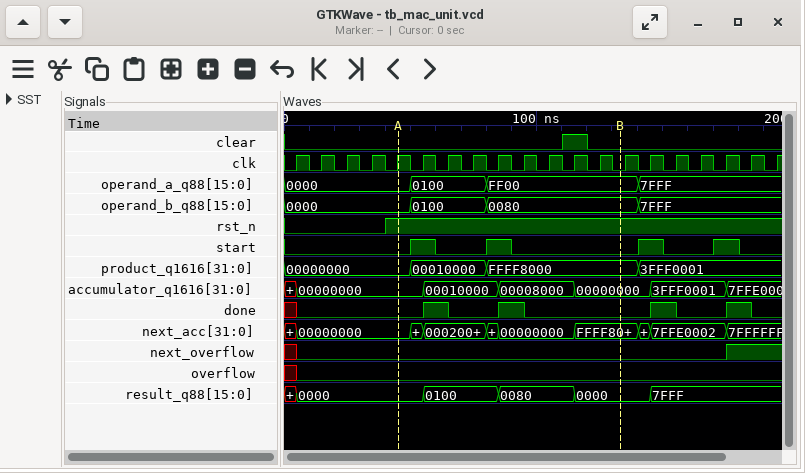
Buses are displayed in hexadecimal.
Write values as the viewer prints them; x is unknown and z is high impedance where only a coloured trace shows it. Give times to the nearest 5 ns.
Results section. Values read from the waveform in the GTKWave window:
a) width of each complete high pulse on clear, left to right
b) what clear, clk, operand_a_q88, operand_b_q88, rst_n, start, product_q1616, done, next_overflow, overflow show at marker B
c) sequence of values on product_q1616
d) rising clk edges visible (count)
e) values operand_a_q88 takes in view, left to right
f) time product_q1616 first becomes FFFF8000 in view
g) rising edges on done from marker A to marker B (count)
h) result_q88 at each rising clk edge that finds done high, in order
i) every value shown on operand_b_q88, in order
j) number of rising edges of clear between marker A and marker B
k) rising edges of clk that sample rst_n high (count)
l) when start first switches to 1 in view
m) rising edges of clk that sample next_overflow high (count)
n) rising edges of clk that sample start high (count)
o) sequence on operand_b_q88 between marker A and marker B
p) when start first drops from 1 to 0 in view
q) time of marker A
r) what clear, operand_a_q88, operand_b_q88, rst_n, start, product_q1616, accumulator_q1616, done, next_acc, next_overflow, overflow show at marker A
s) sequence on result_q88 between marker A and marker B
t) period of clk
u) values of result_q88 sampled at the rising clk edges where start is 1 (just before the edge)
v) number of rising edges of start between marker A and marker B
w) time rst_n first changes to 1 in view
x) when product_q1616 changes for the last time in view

10 ns
clear=0, clk=0, operand_a_q88=FF00, operand_b_q88=0080, rst_n=1, start=0, product_q1616=FFFF8000, done=0, next_overflow=0, overflow=0
00000000, 00010000, FFFF8000, 3FFF0001
20
0000, 0100, FF00, 7FFF
80 ns
2
0100, 0080, 7FFF, 7FFF
0000, 0100, 0080, 7FFF
1
16
50 ns
2
4
0000, 0100, 0080
60 ns
45 ns
clear=0, operand_a_q88=0000, operand_b_q88=0000, rst_n=1, start=0, product_q1616=00000000, accumulator_q1616=00000000, done=0, next_acc=00000000, next_overflow=0, overflow=0
0000, 0100, 0080, 0000
10 ns
0000, 0100, 0000, 7FFF
2
40 ns
140 ns
